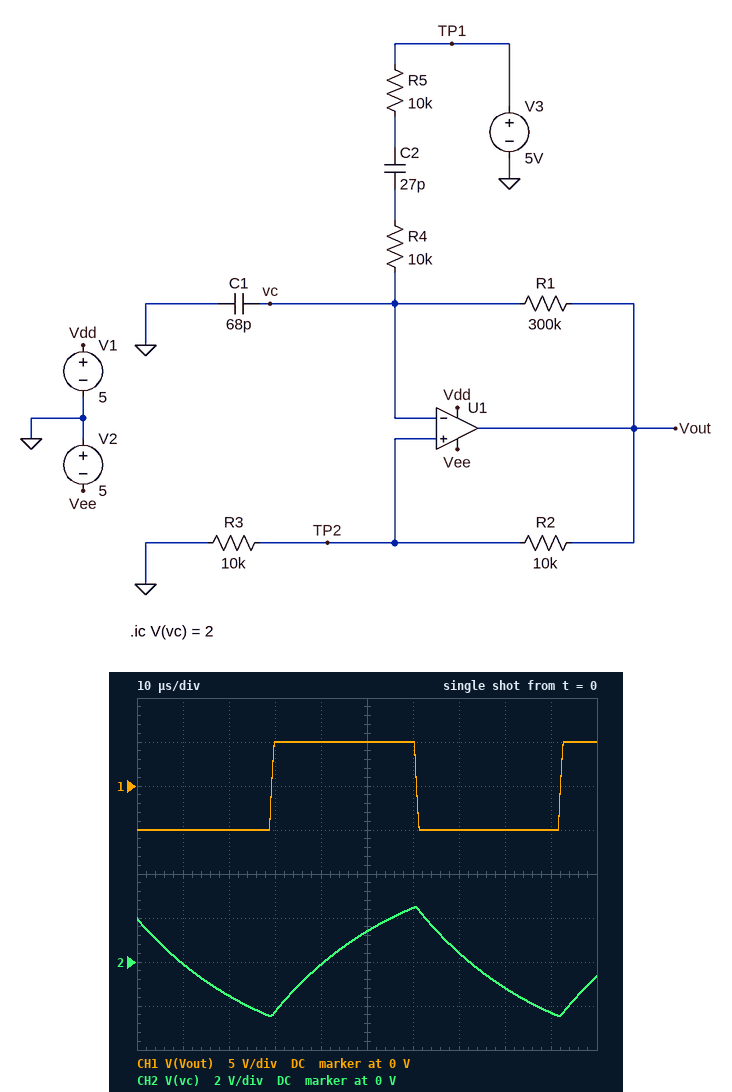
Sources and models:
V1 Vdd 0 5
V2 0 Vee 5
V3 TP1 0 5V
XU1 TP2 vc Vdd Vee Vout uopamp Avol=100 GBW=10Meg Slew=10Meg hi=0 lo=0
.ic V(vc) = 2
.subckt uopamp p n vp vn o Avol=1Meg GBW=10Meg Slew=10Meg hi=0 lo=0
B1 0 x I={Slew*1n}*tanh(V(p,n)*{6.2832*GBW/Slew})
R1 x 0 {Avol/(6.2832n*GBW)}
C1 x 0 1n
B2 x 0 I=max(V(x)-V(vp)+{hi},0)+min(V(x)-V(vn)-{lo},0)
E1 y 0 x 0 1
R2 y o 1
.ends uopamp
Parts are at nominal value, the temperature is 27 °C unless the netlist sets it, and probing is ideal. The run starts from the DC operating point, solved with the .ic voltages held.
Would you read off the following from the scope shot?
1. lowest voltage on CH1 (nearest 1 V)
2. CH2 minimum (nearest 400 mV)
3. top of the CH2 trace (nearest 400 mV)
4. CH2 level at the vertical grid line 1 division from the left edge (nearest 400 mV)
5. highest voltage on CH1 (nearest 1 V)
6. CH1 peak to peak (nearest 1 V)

-5 V
-2.4 V
2.4 V
0 V
5 V
10 V
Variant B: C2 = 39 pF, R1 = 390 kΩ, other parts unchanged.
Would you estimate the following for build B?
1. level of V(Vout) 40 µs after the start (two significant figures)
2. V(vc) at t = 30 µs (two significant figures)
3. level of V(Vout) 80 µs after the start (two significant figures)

-5.0 V
-1.6 V
5.0 V
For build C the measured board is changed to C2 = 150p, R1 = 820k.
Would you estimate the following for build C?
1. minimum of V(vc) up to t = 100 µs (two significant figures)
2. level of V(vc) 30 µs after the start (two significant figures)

-1.0 V
860 mV
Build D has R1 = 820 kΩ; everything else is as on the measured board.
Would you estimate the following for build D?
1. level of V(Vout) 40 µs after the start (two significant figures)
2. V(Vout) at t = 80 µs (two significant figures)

-5.0 V
5.0 V
